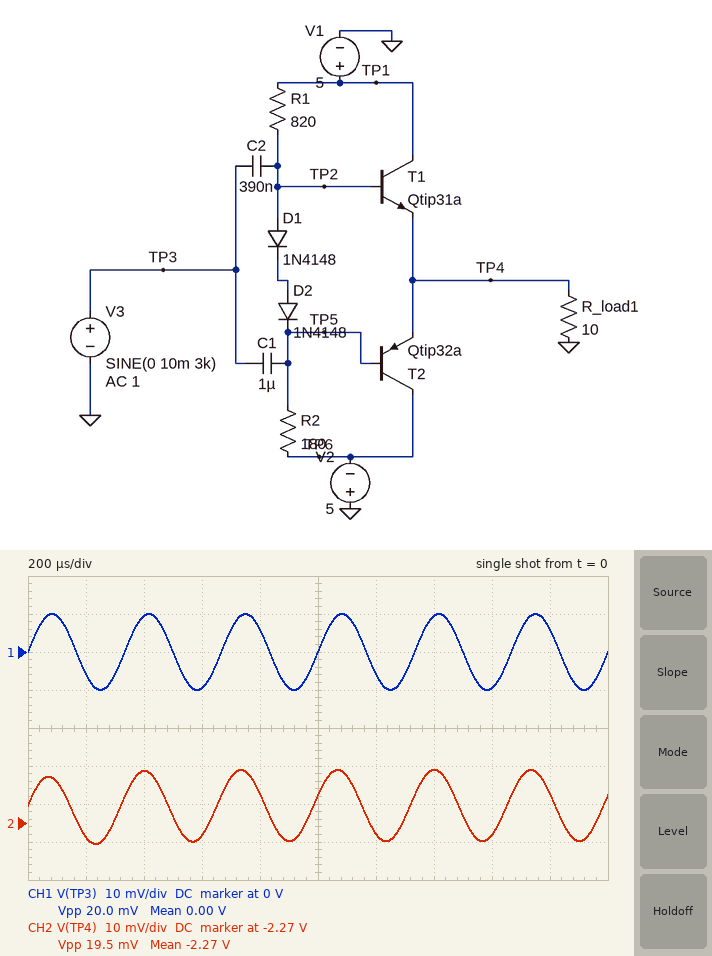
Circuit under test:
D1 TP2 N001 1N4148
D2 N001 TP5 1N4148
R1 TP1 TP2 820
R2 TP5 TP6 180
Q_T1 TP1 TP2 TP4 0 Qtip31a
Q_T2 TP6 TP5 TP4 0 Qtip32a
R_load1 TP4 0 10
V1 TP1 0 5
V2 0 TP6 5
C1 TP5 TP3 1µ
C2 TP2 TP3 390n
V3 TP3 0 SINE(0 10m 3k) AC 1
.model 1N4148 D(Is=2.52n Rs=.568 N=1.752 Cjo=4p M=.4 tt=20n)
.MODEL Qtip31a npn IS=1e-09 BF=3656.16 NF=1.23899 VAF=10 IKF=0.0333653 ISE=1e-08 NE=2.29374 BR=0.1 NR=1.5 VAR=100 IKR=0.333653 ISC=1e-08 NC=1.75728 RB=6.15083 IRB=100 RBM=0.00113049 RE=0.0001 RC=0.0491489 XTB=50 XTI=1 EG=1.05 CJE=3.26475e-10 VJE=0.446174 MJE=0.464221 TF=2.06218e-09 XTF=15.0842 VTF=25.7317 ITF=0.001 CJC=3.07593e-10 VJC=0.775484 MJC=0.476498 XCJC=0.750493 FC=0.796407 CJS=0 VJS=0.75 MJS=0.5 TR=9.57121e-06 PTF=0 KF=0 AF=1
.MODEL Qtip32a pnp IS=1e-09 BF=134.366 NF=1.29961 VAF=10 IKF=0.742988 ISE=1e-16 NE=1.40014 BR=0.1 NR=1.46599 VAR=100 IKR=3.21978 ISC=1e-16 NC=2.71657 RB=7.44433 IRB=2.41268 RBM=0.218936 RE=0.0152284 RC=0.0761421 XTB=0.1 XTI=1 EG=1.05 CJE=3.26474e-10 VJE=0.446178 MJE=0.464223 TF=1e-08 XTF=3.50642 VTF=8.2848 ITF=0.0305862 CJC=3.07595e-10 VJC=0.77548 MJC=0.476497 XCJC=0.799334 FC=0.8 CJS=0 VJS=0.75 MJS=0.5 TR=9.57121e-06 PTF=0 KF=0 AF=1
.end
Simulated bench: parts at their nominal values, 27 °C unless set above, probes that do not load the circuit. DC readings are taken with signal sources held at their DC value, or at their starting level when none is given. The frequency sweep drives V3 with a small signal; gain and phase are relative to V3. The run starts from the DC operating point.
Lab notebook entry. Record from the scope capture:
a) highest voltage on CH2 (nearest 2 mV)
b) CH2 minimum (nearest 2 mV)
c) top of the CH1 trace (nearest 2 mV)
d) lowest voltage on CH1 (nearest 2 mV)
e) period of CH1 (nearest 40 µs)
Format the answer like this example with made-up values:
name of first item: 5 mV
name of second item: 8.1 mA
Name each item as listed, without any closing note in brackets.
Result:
highest voltage on CH2: -2.256 V
CH2 minimum: -2.276 V
top of the CH1 trace: 10 mV
lowest voltage on CH1: -10 mV
period of CH1: 320 µs
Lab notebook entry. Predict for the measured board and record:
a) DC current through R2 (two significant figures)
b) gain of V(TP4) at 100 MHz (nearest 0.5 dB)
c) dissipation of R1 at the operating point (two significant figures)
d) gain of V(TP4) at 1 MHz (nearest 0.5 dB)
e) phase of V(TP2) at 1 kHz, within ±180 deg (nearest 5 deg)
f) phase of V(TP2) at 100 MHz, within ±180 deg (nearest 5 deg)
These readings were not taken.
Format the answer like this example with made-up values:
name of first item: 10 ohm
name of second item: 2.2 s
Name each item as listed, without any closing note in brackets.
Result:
DC current through R2: 11 mA
gain of V(TP4) at 100 MHz: -3.5 dB
dissipation of R1 at the operating point: 53 mW
gain of V(TP4) at 1 MHz: -0.5 dB
phase of V(TP2) at 1 kHz, within ±180 deg: 40 deg
phase of V(TP2) at 100 MHz, within ±180 deg: 0 deg
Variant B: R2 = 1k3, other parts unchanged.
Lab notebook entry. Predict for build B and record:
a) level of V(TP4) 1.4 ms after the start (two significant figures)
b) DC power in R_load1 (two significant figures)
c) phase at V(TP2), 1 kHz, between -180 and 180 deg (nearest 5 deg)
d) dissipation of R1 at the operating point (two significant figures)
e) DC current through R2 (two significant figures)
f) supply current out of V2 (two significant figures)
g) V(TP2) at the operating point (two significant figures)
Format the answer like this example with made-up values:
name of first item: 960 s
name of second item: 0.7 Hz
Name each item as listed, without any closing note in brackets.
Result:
level of V(TP4) 1.4 ms after the start: 850 mV
DC power in R_load1: 71 mW
phase at V(TP2), 1 kHz, between -180 and 180 deg: 15 deg
dissipation of R1 at the operating point: 15 mW
DC current through R2: 4.0 mA
supply current out of V2: 120 mA
V(TP2) at the operating point: 1.5 V
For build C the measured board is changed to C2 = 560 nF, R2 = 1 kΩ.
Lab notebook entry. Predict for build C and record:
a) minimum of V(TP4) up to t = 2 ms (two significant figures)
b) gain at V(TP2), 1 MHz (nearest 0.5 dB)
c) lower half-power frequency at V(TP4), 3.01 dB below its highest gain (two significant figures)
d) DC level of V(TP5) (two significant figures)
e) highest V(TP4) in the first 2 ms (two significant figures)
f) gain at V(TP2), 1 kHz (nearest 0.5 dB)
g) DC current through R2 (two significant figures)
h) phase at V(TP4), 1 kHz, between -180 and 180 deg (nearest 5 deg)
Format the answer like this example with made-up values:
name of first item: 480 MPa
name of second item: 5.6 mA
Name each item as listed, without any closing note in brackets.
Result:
minimum of V(TP4) up to t = 2 ms: 430 mV
gain at V(TP2), 1 MHz: 0 dB
lower half-power frequency at V(TP4), 3.01 dB below its highest gain: 300 Hz
DC level of V(TP5): -190 mV
highest V(TP4) in the first 2 ms: 450 mV
gain at V(TP2), 1 kHz: -0.5 dB
DC current through R2: 4.8 mA
phase at V(TP4), 1 kHz, between -180 and 180 deg: 15 deg
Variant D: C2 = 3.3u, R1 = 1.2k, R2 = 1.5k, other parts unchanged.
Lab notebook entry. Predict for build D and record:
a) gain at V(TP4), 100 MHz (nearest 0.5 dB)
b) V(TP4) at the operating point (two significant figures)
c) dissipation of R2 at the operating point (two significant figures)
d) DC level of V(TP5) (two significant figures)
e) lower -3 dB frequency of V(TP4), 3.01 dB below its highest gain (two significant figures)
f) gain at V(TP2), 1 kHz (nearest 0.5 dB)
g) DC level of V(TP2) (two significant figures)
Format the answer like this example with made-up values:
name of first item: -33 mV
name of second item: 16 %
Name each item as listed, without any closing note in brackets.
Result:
gain at V(TP4), 100 MHz: -3.0 dB
V(TP4) at the operating point: 450 mV
dissipation of R2 at the operating point: 16 mW
DC level of V(TP5): -160 mV
lower -3 dB frequency of V(TP4), 3.01 dB below its highest gain: 77 Hz
gain at V(TP2), 1 kHz: 0 dB
DC level of V(TP2): 1.1 V
